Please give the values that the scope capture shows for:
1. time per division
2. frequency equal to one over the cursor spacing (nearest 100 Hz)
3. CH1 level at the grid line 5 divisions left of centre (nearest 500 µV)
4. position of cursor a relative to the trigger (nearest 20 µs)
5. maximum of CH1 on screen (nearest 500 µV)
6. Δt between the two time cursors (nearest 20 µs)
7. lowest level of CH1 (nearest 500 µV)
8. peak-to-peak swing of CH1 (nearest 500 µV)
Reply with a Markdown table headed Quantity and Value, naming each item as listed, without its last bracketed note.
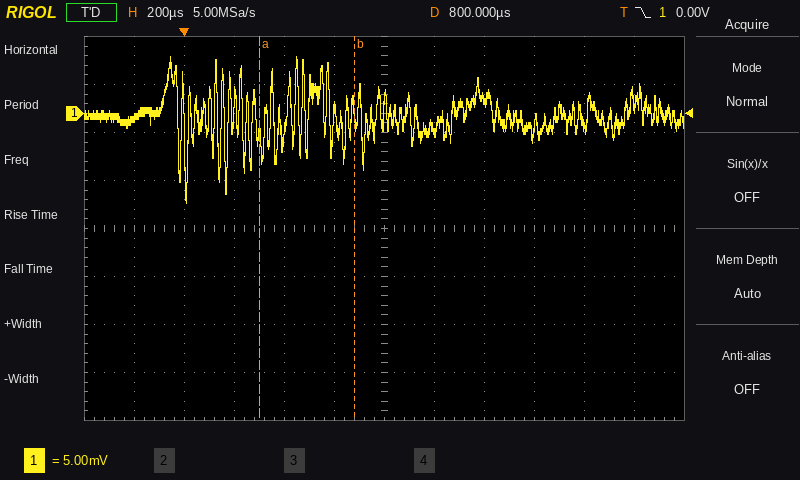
| Quantity | Value |
|---|---|
| time per division | 200 µs |
| frequency equal to one over the cursor spacing | 2.6 kHz |
| CH1 level at the grid line 5 divisions left of centre | -500 µV |
| position of cursor a relative to the trigger | +300 µs |
| maximum of CH1 on screen | 6.0 mV |
| Δt between the two time cursors | 380 µs |
| lowest level of CH1 | -9.5 mV |
| peak-to-peak swing of CH1 | 15.5 mV |
